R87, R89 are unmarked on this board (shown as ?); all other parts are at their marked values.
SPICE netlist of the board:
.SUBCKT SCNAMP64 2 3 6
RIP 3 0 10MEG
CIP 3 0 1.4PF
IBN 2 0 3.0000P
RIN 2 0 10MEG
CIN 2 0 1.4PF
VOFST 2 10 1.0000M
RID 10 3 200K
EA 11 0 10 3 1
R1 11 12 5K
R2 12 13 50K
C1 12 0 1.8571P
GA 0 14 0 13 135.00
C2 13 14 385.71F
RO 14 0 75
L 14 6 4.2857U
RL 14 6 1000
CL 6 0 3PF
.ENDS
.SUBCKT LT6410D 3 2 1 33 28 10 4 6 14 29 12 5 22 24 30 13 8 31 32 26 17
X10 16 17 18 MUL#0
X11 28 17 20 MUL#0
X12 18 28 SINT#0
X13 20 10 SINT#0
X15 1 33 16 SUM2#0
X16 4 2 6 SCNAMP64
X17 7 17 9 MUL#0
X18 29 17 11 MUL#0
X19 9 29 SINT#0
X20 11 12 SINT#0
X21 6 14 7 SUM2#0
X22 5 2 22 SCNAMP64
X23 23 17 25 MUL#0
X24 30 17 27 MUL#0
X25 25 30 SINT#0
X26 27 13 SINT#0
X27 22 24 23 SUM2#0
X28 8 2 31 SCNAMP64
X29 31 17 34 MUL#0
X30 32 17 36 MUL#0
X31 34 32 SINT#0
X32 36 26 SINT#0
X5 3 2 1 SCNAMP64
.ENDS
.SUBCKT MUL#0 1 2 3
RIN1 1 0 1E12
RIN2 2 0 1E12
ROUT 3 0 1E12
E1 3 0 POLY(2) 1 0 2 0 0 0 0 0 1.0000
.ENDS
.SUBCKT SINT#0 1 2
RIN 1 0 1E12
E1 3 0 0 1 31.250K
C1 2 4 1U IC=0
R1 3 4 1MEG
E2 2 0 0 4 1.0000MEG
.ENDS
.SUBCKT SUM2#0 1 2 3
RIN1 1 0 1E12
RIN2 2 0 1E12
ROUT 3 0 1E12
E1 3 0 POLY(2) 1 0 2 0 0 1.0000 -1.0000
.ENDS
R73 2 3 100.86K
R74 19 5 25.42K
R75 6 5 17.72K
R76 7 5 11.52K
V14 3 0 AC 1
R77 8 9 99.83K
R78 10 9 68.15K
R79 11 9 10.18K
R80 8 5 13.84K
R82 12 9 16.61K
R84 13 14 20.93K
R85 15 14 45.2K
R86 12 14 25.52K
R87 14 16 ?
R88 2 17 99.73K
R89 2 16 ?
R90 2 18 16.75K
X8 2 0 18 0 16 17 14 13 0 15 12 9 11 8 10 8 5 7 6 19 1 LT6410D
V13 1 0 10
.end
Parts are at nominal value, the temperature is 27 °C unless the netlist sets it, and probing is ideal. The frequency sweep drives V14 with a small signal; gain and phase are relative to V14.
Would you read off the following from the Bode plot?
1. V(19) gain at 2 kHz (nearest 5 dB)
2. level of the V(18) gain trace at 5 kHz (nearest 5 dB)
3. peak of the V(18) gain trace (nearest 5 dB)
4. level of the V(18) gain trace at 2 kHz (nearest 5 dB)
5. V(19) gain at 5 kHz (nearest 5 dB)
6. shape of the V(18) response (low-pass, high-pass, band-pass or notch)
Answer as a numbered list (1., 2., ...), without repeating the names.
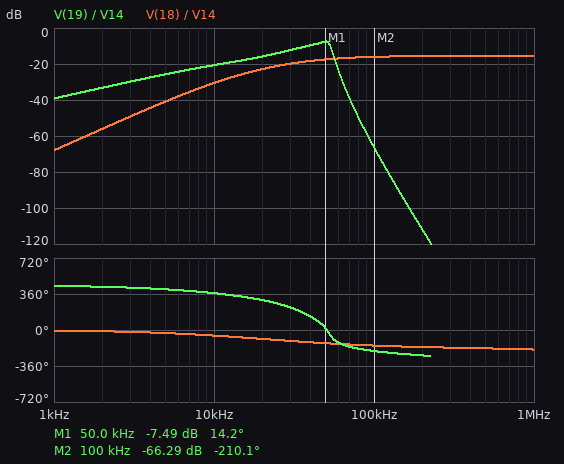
1. -35 dB
2. -40 dB
3. -15 dB
4. -55 dB
5. -25 dB
6. high-pass
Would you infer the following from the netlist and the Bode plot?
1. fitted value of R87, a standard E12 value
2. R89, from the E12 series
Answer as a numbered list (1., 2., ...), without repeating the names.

1. 47 kΩ
2. 18 kΩ
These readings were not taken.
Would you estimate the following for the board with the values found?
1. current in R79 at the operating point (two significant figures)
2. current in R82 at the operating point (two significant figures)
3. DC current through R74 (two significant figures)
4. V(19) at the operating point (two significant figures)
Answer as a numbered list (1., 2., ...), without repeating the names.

1. 110 nA
2. 140 nA
3. 230 nA
4. 6.8 mV
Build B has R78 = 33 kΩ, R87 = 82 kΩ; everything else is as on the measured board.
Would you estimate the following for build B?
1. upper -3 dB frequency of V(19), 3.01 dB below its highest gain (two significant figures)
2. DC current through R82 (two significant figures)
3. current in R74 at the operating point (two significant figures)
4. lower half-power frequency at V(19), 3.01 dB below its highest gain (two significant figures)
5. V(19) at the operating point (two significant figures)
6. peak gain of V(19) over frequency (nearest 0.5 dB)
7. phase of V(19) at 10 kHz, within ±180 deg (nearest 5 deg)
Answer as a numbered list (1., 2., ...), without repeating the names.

1. 51 kHz
2. 130 nA
3. 210 nA
4. 27 kHz
5. 6.3 mV
6. -15.0 dB
7. 5 deg
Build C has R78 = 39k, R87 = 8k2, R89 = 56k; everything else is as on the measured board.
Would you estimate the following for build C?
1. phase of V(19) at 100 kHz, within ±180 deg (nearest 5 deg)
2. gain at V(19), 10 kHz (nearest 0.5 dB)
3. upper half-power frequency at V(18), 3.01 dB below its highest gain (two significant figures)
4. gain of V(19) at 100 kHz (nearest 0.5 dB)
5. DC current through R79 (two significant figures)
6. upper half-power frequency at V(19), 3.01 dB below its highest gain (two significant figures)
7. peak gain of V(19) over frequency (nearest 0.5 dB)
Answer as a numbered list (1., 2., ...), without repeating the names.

1. 135 deg
2. -1.5 dB
3. 84 kHz
4. -50.5 dB
5. 240 nA
6. 50 kHz
7. 10.0 dB
